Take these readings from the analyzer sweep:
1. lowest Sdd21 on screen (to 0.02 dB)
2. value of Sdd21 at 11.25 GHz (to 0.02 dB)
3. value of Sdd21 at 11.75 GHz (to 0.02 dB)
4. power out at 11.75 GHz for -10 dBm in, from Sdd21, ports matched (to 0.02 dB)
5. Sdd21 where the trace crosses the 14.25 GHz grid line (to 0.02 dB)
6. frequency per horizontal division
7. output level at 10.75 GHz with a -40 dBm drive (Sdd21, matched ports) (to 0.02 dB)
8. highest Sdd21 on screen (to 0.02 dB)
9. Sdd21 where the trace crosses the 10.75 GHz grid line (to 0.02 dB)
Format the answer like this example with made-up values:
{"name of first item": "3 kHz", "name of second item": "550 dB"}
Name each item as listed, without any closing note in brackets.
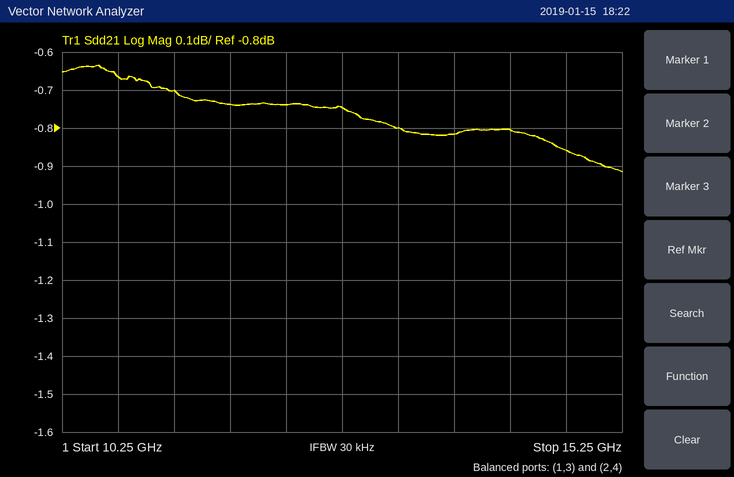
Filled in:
{"lowest Sdd21 on screen": "-0.92 dB", "value of Sdd21 at 11.25 GHz": "-0.70 dB", "value of Sdd21 at 11.75 GHz": "-0.74 dB", "power out at 11.75 GHz for -10 dBm in, from Sdd21, ports matched": "-10.74 dBm", "Sdd21 where the trace crosses the 14.25 GHz grid line": "-0.80 dB", "frequency per horizontal division": "500 MHz", "output level at 10.75 GHz with a -40 dBm drive (Sdd21, matched ports)": "-40.66 dBm", "highest Sdd21 on screen": "-0.64 dB", "Sdd21 where the trace crosses the 10.75 GHz grid line": "-0.66 dB"}
